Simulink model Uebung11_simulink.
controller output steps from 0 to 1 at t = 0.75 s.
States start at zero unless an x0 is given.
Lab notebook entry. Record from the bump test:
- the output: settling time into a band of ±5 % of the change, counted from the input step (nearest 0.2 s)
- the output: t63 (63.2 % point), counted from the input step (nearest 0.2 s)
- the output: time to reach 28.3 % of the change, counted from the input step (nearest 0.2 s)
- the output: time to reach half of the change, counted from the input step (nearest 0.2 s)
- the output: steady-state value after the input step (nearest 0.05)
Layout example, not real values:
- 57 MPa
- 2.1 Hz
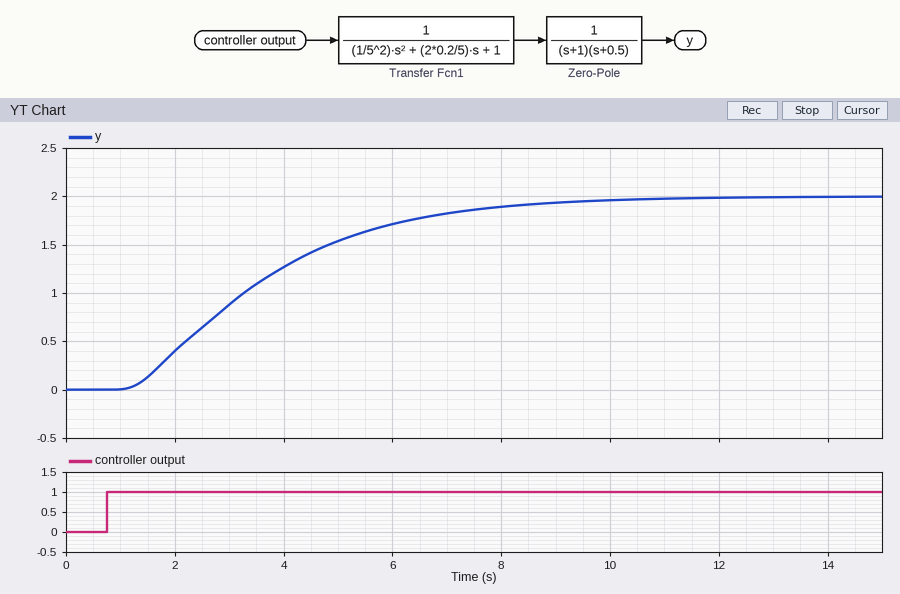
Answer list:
- 7.4 s
- 3.2 s
- 1.6 s
- 2.6 s
- 2.00
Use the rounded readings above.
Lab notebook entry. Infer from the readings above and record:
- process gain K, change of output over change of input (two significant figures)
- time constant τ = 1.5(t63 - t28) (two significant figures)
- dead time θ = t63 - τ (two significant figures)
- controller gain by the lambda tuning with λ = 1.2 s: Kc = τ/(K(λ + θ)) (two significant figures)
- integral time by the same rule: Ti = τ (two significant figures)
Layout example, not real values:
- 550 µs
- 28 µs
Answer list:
- 2.0
- 2.4 s
- 0.80 s
- 0.60
- 2.4 s
